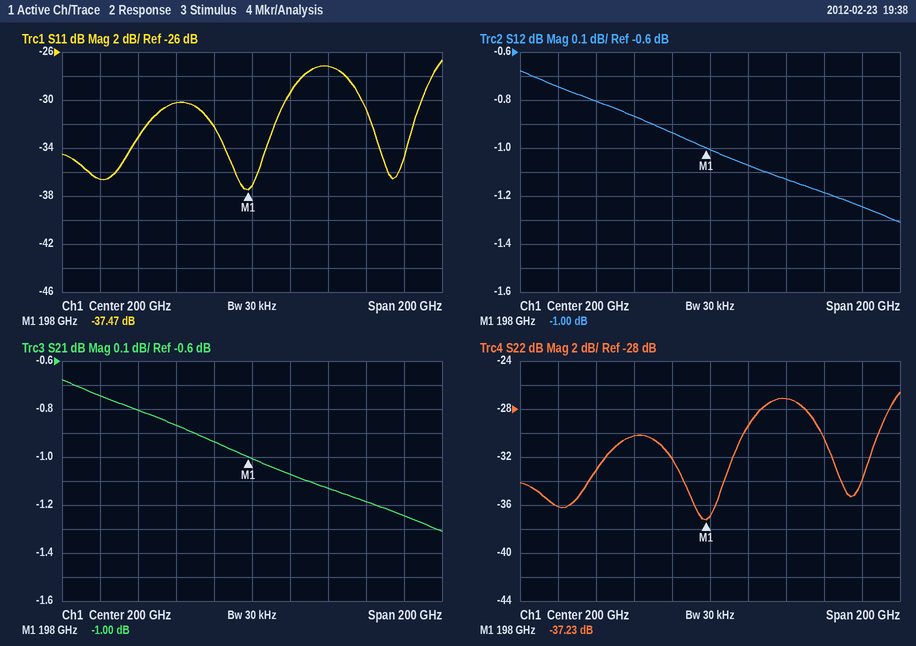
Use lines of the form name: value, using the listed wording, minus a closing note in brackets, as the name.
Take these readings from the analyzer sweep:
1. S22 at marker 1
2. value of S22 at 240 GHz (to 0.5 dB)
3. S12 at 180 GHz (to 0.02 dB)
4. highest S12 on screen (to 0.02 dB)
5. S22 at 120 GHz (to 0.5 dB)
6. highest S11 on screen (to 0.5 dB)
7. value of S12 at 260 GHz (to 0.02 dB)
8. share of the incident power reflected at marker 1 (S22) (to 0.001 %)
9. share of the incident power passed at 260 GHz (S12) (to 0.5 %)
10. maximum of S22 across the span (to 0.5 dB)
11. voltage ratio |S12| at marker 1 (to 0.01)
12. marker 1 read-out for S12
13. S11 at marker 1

S22 at marker 1: -37.23 dB
value of S22 at 240 GHz: -27.0 dB
S12 at 180 GHz: -0.94 dB
highest S12 on screen: -0.68 dB
S22 at 120 GHz: -36.0 dB
highest S11 on screen: -26.5 dB
value of S12 at 260 GHz: -1.18 dB
share of the incident power reflected at marker 1 (S22): 0.019 %
share of the incident power passed at 260 GHz (S12): 76.0 %
maximum of S22 across the span: -26.5 dB
voltage ratio |S12| at marker 1: 0.89
marker 1 read-out for S12: -1.00 dB
S11 at marker 1: -37.47 dB
